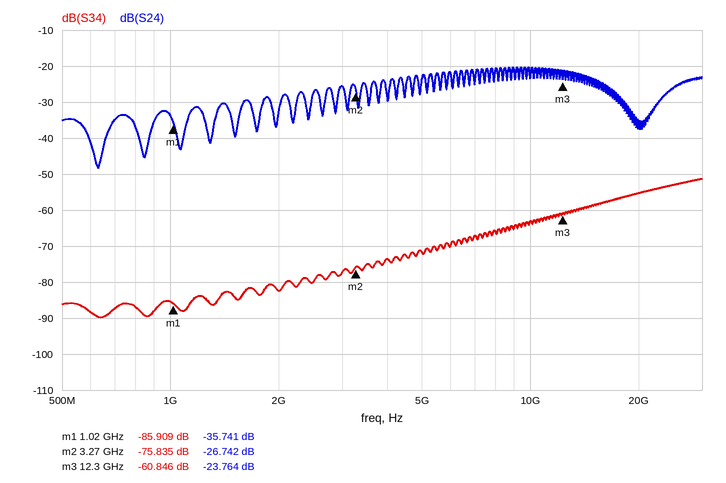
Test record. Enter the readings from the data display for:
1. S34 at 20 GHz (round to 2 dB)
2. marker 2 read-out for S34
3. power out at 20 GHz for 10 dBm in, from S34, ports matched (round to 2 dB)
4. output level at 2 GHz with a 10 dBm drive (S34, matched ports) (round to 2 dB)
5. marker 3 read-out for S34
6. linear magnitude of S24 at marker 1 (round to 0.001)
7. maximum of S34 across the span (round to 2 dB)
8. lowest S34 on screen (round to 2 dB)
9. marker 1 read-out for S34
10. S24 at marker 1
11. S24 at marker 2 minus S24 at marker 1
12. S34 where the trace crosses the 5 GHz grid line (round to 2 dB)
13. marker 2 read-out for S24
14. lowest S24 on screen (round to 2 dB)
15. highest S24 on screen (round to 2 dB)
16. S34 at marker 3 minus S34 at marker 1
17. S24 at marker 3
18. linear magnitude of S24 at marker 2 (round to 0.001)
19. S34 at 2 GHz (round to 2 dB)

-56 dB
-75.835 dB
-46 dBm
-72 dBm
-60.846 dB
0.016
-52 dB
-90 dB
-85.909 dB
-35.741 dB
8.999 dB
-72 dB
-26.742 dB
-48 dB
-20 dB
25.063 dB
-23.764 dB
0.046
-82 dB
